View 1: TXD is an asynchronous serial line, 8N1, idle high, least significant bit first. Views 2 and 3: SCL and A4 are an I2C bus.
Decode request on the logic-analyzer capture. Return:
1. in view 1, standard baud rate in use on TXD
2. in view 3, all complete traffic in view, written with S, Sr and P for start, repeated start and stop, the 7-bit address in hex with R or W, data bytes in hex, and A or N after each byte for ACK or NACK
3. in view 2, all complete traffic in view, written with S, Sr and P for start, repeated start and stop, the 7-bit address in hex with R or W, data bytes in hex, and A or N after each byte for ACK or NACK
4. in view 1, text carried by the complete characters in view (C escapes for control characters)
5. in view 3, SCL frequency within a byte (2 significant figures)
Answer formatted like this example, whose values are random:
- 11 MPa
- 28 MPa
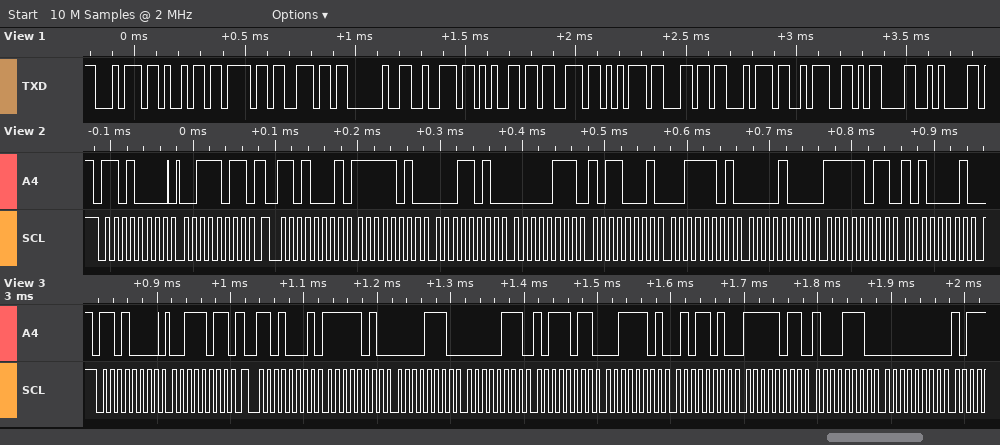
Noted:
- 38400 baud
- S 68W A 3B A Sr 68R A FA A 0E A 07 A BB A 3D A 5A A FB A 8E A 00 A
- S 68W A 3B A Sr 68R A FA A 1A A 07 A B1 A 3D A 08 A FB A A1 A
- "tion result:\r\n"
- 100 kHz
